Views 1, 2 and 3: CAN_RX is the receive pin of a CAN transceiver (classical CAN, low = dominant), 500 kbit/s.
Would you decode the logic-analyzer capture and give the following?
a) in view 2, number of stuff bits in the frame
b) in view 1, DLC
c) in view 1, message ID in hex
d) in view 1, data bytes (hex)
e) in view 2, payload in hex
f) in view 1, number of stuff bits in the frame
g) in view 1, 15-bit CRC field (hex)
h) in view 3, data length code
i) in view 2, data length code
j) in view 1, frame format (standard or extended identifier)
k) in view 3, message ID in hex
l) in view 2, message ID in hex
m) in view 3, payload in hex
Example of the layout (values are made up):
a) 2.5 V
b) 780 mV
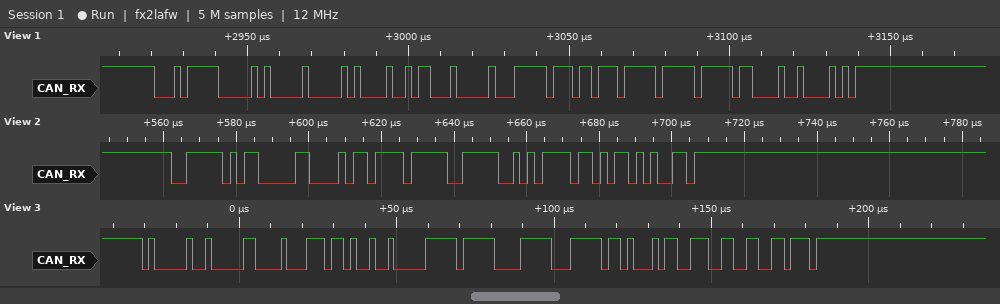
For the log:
a) 4
b) 8
c) 0x17C
d) 00 84 B1 00 FF 6E FF FF
e) 2D EF BE AF
f) 9
g) 0x4242
h) 8
i) 4
j) standard
k) 0x404
l) 0x3F6
m) 47 69 20 FF 8F 9F D1 67
